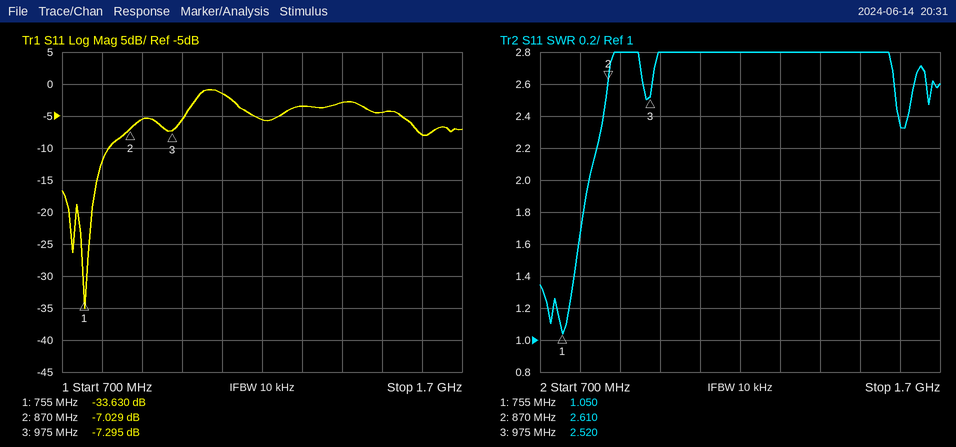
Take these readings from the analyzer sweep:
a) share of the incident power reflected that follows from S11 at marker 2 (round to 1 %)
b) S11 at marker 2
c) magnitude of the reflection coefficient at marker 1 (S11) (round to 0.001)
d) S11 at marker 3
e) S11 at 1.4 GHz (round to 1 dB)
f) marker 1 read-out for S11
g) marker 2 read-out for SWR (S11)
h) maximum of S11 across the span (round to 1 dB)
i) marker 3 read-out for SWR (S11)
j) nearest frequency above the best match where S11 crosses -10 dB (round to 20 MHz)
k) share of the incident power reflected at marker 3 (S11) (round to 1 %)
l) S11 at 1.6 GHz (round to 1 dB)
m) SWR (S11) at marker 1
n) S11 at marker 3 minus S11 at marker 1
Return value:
20 %
-7.029 dB
0.021
-7.295 dB
-3 dB
-33.630 dB
2.610
-1 dB
2.520
820 MHz
19 %
-8 dB
1.050
26.335 dB
